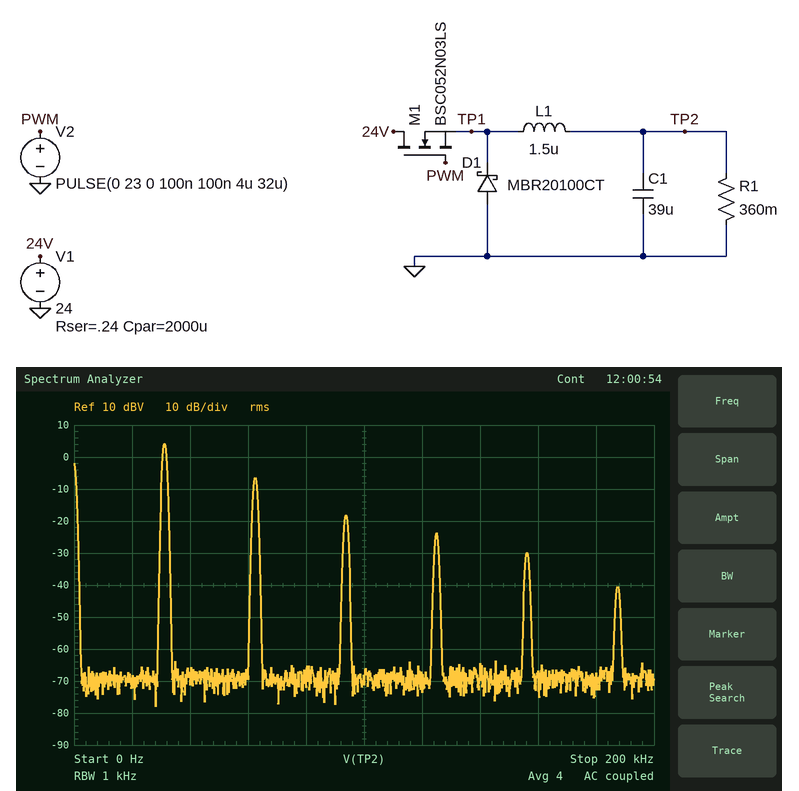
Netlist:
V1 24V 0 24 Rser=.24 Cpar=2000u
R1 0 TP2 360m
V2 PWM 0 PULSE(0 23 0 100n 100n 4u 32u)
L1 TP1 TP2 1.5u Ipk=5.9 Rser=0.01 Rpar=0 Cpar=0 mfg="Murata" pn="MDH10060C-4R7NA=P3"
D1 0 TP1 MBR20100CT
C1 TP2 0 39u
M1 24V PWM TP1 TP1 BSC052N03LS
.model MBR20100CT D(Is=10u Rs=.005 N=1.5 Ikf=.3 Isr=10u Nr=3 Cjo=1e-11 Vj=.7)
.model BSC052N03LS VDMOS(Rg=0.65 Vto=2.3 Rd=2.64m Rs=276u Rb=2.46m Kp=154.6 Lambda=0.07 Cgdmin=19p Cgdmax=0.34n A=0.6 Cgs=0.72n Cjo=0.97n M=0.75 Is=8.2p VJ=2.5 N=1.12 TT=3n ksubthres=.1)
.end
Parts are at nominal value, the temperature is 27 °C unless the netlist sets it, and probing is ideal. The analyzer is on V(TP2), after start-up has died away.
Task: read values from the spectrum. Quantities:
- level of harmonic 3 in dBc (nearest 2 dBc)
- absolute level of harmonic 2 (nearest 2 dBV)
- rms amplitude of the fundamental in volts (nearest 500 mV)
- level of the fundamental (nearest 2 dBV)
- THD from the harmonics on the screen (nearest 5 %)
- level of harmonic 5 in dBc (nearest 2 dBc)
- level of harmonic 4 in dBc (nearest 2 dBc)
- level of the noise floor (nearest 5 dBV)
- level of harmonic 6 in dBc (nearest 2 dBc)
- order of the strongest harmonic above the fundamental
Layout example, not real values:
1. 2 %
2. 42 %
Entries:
1. -22 dBc
2. -6 dBV
3. 1.5 V
4. 4 dBV
5. 30 %
6. -34 dBc
7. -28 dBc
8. -70 dBV
9. -44 dBc
10. 2
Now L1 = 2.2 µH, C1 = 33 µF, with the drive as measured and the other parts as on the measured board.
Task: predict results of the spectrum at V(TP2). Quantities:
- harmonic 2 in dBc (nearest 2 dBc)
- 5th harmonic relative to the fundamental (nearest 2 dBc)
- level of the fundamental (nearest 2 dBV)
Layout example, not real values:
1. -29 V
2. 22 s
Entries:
1. -12 dBc
2. -36 dBc
3. 4 dBV
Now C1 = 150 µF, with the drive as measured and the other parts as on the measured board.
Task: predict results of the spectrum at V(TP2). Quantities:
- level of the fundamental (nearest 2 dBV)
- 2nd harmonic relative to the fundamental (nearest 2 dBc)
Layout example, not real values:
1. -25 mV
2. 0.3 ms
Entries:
1. -8 dBV
2. -12 dBc
